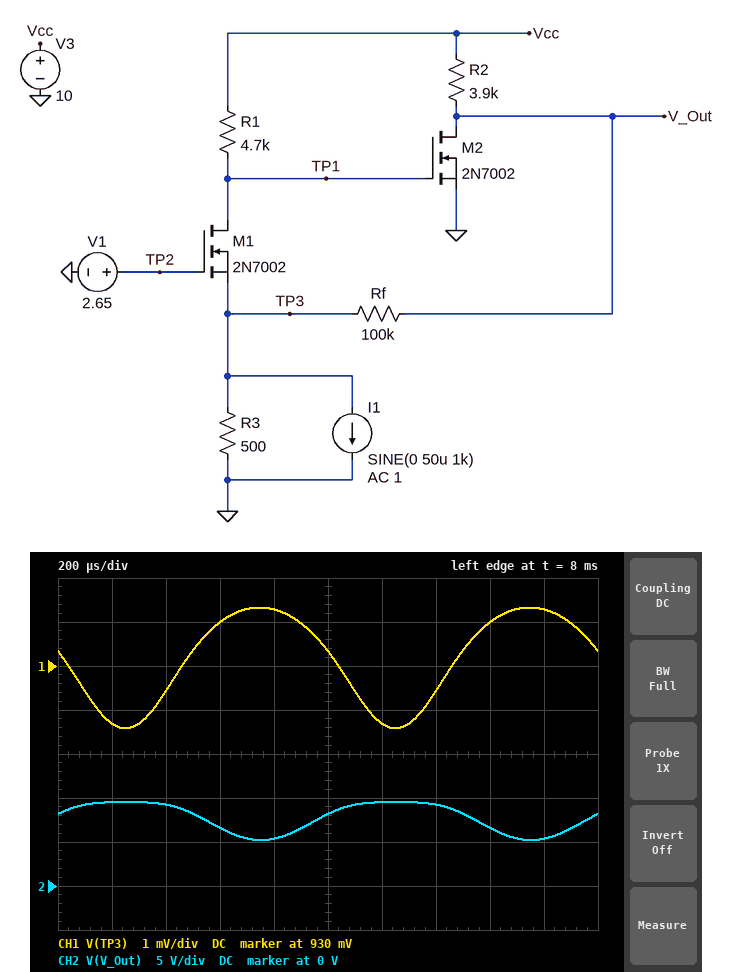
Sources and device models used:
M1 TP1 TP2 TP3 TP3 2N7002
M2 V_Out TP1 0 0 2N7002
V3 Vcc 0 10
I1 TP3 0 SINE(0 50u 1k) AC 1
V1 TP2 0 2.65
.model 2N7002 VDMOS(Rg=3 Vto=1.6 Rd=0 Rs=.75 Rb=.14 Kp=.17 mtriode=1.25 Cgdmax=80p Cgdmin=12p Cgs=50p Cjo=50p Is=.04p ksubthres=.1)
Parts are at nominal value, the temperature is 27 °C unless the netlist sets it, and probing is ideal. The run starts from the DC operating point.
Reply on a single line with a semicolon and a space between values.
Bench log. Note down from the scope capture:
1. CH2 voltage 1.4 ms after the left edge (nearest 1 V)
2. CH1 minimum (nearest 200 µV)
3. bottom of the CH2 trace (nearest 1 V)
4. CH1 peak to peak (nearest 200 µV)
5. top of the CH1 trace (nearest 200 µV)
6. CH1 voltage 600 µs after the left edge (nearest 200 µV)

9 V; 928.6 mV; 5 V; 2.8 mV; 931.4 mV; 931.0 mV
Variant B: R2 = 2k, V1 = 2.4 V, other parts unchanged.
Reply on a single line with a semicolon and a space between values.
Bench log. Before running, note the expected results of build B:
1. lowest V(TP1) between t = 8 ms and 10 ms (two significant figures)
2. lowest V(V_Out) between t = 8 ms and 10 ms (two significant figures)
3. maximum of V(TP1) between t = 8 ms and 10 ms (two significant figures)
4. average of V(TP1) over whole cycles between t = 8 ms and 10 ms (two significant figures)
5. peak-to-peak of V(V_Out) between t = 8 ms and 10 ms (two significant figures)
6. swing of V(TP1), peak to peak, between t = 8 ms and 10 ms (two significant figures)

3.2 V; 16 mV; 3.6 V; 3.4 V; 3.2 mV; 420 mV
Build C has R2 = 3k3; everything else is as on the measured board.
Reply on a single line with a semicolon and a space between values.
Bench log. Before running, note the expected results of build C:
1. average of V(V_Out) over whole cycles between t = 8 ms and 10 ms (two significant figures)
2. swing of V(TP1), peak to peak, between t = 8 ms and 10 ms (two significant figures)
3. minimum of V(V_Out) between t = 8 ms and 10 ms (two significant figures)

7.9 V; 250 mV; 5.5 V
